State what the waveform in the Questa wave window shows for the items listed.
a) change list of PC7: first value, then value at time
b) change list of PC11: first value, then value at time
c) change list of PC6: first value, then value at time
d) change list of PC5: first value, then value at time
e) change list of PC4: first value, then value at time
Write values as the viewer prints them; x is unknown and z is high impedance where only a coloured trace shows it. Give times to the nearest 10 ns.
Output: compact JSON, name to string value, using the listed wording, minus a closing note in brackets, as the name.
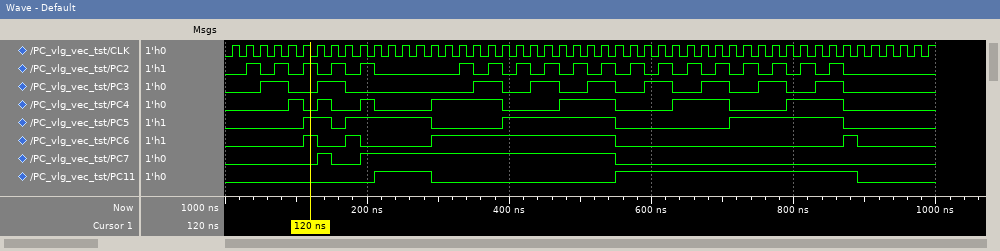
{"change list of PC7: first value, then value at time": "0, 1 at 130 ns, 0 at 150 ns, 1 at 190 ns, 0 at 550 ns", "change list of PC11: first value, then value at time": "0, 1 at 210 ns, 0 at 290 ns, 1 at 550 ns, 0 at 890 ns", "change list of PC6: first value, then value at time": "0, 1 at 110 ns, 0 at 130 ns, 1 at 170 ns, 0 at 190 ns, 1 at 290 ns, 0 at 550 ns, 1 at 870 ns, 0 at 890 ns", "change list of PC5: first value, then value at time": "0, 1 at 110 ns, 0 at 150 ns, 1 at 170 ns, 0 at 290 ns, 1 at 390 ns, 0 at 550 ns, 1 at 710 ns, 0 at 870 ns", "change list of PC4: first value, then value at time": "0, 1 at 90 ns, 0 at 110 ns, 1 at 130 ns, 0 at 150 ns, 1 at 190 ns, 0 at 210 ns, 1 at 290 ns, 0 at 390 ns, 1 at 470 ns, 0 at 550 ns, 1 at 630 ns, 0 at 710 ns, 1 at 790 ns, 0 at 870 ns"}
